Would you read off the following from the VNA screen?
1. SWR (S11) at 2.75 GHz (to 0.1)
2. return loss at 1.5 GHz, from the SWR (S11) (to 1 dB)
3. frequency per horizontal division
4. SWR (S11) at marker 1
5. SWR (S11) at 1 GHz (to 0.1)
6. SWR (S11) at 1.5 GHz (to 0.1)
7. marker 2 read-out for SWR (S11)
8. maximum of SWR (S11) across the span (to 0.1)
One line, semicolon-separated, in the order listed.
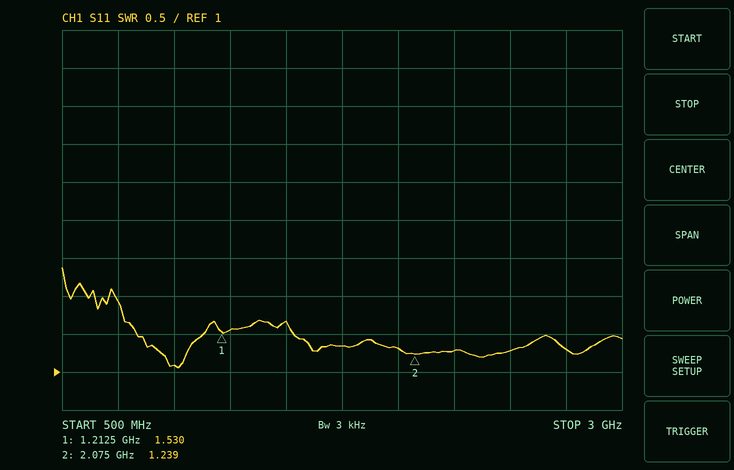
1.3; 12 dB; 250 MHz; 1.530; 1.1; 1.7; 1.239; 2.4
